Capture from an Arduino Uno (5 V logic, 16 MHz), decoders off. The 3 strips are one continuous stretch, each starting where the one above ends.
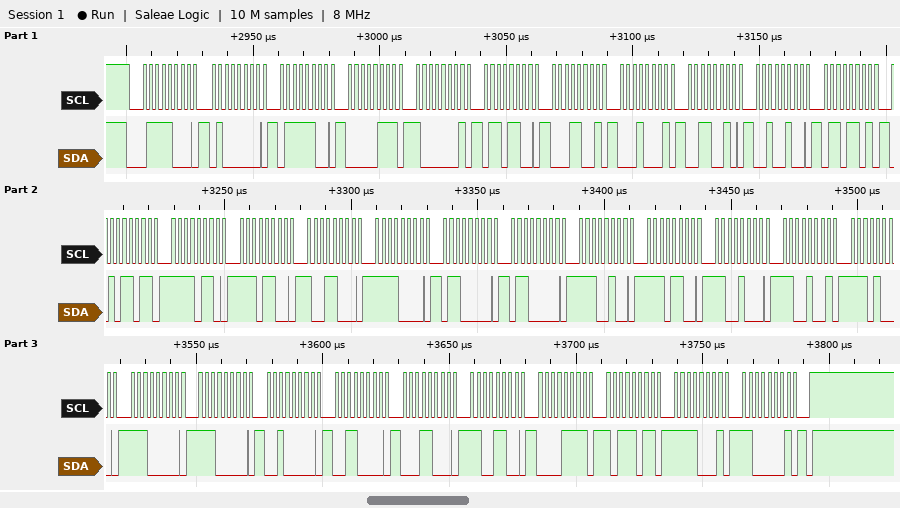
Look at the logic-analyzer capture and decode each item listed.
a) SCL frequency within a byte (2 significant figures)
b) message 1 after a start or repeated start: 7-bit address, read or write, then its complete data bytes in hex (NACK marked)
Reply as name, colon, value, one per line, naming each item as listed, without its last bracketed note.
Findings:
SCL frequency within a byte: 400 kHz
message 1 after a start or repeated start: 7-bit address, read or write, then its complete data bytes in hex: 0x3C write: 40 7C 07 81 6C 19 11 32 24 6D 5B F6 EC 98 F0 60 60 E4 EC C8 C9 E8 E0 E0 20 30 18 CC 0F BB F1 C1
